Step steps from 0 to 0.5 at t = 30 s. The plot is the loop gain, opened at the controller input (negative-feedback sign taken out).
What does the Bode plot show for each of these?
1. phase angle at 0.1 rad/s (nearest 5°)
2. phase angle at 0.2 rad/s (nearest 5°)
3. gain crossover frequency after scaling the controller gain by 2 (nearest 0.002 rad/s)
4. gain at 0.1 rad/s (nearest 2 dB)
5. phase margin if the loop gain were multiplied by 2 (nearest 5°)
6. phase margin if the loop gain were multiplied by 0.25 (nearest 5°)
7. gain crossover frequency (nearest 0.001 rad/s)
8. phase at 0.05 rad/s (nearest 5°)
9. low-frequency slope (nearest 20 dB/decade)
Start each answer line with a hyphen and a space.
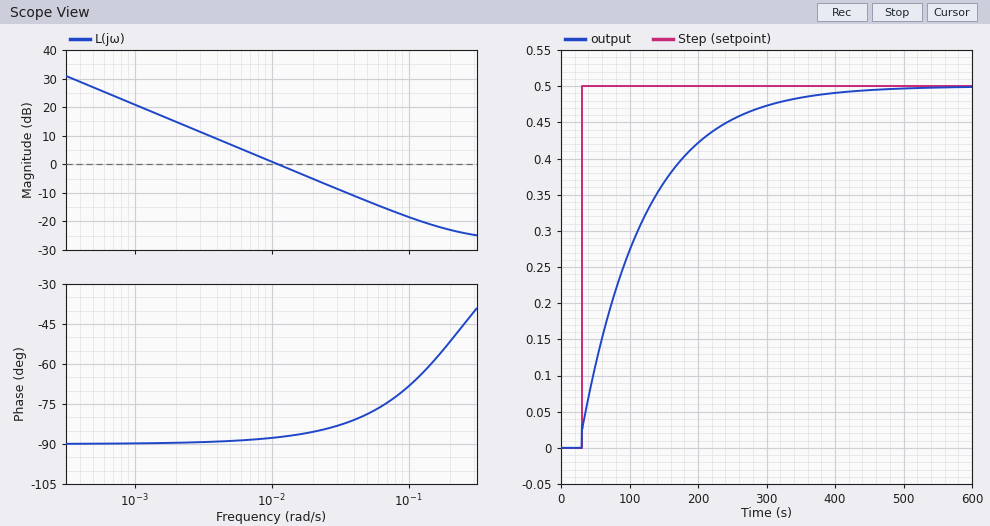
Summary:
- -70°
- -50°
- 0.022 rad/s
- -18 dB
- 95°
- 90°
- 0.011 rad/s
- -80°
- -20 dB/decade
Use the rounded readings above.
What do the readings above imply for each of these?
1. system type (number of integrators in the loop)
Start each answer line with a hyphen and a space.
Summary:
- 1
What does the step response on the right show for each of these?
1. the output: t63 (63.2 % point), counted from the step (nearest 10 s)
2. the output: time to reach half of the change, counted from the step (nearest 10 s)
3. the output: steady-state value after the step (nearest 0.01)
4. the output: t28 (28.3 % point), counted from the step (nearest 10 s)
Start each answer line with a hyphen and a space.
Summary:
- 90 s
- 60 s
- 0.50
- 30 s
